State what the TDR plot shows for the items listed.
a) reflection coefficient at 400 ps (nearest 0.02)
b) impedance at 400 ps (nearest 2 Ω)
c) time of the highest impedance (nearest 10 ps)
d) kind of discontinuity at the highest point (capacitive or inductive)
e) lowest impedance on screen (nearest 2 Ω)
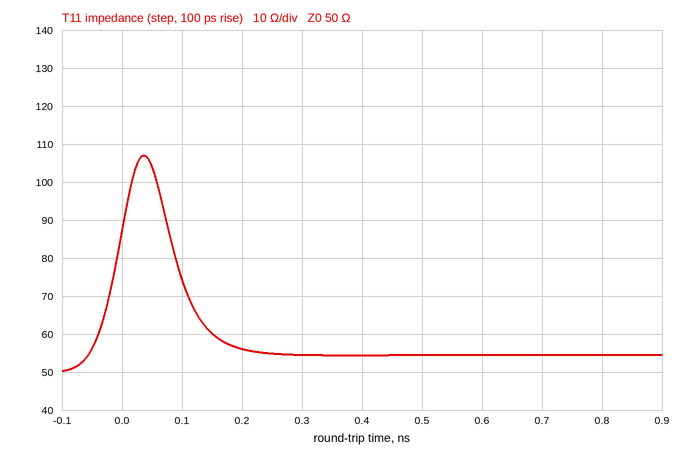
+0.04
54 Ω
40 ps
inductive
50 Ω
